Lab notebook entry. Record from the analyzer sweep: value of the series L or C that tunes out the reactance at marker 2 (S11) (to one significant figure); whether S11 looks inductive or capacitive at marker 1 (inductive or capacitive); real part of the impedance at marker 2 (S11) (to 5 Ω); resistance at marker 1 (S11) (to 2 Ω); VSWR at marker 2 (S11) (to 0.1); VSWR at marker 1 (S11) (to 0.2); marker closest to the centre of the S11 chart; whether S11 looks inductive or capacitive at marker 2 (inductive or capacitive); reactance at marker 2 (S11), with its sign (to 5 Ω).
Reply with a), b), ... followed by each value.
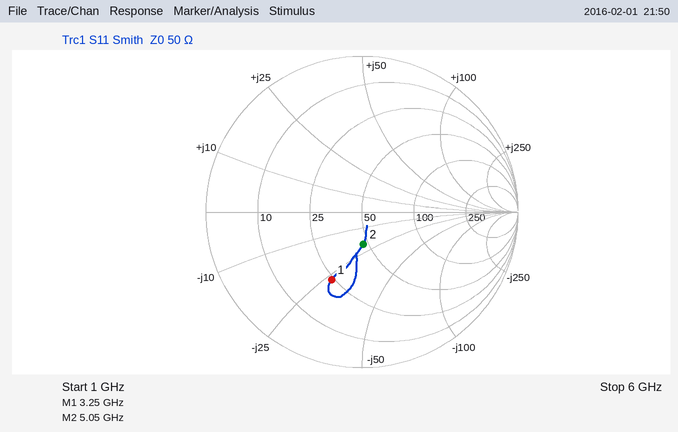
a) 600 pH
b) capacitive
c) 45 Ω
d) 24 Ω
e) 1.5
f) 2.8
g) marker 2
h) capacitive
i) -20 Ω
